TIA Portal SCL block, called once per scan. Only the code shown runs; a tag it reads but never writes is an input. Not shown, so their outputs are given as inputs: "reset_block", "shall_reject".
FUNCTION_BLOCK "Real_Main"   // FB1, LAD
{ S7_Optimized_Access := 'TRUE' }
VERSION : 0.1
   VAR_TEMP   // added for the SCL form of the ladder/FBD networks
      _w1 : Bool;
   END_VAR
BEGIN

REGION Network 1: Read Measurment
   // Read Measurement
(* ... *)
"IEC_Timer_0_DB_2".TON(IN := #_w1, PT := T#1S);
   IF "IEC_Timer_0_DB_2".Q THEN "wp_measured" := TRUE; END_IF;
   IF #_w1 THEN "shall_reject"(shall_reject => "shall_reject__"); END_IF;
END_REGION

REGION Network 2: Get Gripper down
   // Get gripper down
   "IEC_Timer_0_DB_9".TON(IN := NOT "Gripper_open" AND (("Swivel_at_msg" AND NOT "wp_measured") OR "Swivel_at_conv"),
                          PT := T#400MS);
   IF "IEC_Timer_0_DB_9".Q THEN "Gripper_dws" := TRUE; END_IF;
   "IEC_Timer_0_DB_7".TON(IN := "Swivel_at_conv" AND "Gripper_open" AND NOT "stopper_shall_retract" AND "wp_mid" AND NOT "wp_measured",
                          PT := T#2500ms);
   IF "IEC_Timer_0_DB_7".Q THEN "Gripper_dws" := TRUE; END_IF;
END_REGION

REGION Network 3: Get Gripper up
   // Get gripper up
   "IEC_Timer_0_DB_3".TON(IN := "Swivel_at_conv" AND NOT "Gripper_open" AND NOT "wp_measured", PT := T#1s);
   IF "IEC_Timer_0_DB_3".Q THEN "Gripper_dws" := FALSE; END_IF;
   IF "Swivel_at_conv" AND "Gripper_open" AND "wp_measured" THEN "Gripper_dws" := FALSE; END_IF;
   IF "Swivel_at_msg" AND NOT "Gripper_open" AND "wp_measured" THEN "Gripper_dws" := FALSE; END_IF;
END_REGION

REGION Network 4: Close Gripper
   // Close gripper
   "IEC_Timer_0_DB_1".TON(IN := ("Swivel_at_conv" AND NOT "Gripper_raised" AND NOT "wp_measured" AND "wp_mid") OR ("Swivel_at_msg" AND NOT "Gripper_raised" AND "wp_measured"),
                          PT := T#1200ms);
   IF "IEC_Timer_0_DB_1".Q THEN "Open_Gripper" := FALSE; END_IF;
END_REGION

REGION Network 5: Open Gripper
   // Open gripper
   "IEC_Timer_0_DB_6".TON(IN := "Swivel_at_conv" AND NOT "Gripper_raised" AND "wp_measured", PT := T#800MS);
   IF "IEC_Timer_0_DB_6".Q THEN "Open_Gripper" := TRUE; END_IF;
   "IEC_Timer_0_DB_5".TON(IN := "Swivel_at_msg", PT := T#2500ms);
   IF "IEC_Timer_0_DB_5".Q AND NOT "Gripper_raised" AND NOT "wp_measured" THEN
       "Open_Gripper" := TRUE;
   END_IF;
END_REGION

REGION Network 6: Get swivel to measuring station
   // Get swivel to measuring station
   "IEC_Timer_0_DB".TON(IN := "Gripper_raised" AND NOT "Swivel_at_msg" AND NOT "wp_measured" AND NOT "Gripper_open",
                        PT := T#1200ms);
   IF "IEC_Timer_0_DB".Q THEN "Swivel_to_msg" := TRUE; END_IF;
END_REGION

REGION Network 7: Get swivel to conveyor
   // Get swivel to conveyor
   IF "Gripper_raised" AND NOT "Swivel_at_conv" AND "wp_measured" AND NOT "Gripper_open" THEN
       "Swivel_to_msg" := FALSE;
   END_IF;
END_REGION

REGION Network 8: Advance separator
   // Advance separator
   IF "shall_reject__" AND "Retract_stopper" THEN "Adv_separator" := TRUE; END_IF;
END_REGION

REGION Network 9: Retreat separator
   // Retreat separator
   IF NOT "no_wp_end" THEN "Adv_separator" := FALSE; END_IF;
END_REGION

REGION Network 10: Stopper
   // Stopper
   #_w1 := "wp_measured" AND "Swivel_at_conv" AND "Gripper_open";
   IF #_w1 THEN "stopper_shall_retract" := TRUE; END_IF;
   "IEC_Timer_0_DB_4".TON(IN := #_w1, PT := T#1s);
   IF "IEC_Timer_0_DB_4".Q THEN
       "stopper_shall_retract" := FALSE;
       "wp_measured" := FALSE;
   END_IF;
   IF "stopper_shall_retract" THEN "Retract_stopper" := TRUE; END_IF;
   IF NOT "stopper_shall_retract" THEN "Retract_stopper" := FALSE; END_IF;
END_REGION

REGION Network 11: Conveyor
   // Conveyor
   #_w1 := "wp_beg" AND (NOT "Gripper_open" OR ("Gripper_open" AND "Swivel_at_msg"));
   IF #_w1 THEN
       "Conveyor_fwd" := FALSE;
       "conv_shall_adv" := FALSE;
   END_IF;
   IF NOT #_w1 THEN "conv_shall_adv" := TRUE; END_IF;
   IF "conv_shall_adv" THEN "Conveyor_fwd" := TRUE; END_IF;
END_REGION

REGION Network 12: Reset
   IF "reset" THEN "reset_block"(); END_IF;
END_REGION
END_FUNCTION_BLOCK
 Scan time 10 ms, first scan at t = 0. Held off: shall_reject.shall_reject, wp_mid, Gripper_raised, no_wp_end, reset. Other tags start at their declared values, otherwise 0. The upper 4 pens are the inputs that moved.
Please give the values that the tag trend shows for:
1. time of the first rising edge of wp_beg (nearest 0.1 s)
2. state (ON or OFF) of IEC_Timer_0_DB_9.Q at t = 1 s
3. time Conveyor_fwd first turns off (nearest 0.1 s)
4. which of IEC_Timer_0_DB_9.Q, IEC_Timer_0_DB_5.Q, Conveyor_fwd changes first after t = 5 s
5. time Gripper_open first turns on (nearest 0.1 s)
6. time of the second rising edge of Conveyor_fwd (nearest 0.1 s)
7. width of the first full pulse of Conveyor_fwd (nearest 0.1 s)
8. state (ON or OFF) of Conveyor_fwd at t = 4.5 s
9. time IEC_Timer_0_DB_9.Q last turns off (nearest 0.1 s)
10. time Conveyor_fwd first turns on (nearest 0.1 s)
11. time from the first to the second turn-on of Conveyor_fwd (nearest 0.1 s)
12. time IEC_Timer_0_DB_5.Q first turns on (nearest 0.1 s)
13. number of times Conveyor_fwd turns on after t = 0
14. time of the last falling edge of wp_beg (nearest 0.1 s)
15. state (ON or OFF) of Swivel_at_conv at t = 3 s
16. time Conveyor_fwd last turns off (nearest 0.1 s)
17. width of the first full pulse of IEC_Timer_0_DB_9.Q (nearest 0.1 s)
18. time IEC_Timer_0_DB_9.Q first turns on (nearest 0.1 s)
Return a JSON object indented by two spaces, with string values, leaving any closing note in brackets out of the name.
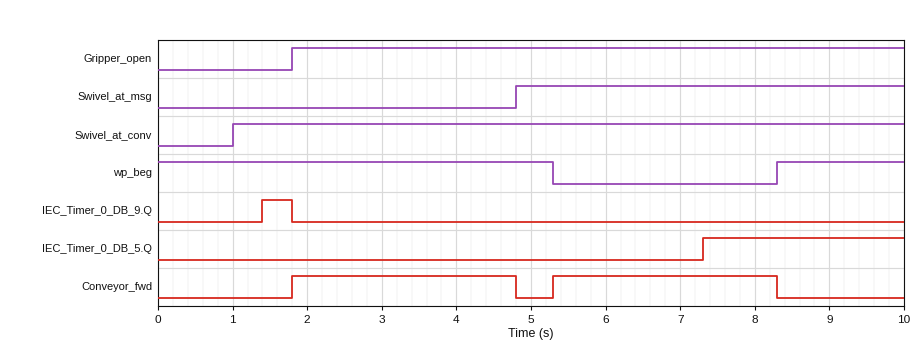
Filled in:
{
  "time of the first rising edge of wp_beg": "8.3 s",
  "state (ON or OFF) of IEC_Timer_0_DB_9.Q at t = 1 s": "OFF",
  "time Conveyor_fwd first turns off": "4.8 s",
  "which of IEC_Timer_0_DB_9.Q, IEC_Timer_0_DB_5.Q, Conveyor_fwd changes first after t = 5 s": "Conveyor_fwd",
  "time Gripper_open first turns on": "1.8 s",
  "time of the second rising edge of Conveyor_fwd": "5.3 s",
  "width of the first full pulse of Conveyor_fwd": "3.0 s",
  "state (ON or OFF) of Conveyor_fwd at t = 4.5 s": "ON",
  "time IEC_Timer_0_DB_9.Q last turns off": "1.8 s",
  "time Conveyor_fwd first turns on": "1.8 s",
  "time from the first to the second turn-on of Conveyor_fwd": "3.5 s",
  "time IEC_Timer_0_DB_5.Q first turns on": "7.3 s",
  "number of times Conveyor_fwd turns on after t = 0": "2",
  "time of the last falling edge of wp_beg": "5.3 s",
  "state (ON or OFF) of Swivel_at_conv at t = 3 s": "ON",
  "time Conveyor_fwd last turns off": "8.3 s",
  "width of the first full pulse of IEC_Timer_0_DB_9.Q": "0.4 s",
  "time IEC_Timer_0_DB_9.Q first turns on": "1.4 s"
}
